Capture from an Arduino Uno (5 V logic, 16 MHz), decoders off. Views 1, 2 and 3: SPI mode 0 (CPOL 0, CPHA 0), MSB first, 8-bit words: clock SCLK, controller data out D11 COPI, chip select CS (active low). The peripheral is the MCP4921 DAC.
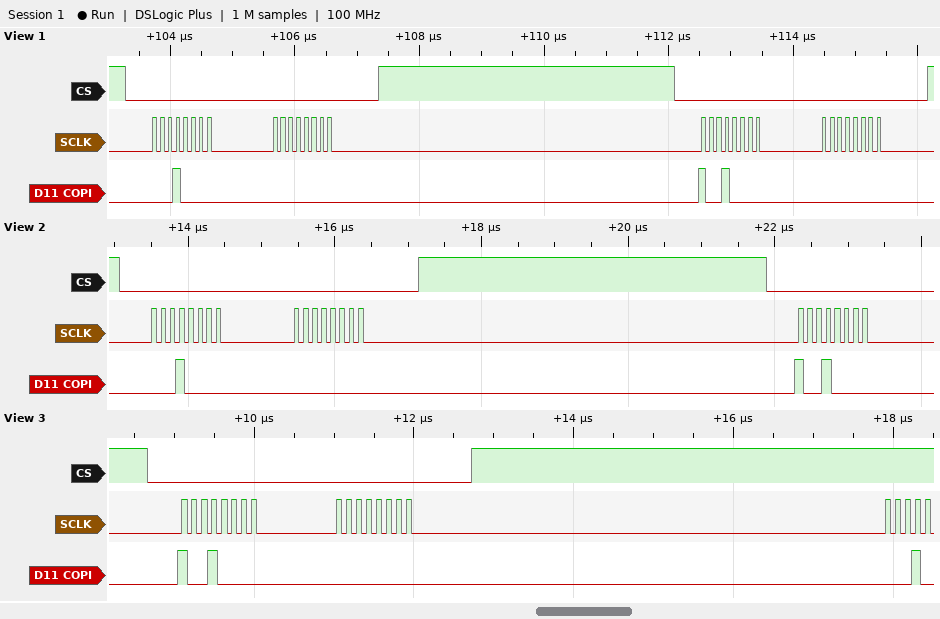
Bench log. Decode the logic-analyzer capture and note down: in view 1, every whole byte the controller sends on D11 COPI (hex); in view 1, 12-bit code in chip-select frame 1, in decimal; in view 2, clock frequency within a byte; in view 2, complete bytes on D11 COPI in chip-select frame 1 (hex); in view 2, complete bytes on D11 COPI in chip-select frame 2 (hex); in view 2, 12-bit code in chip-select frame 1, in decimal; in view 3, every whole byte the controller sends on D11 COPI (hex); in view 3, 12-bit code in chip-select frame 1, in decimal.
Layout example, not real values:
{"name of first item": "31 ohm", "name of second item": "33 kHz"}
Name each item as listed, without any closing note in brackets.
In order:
{"in view 1, every whole byte the controller sends on D11 COPI": "10 00 90 00", "in view 1, 12-bit code in chip-select frame 1, in decimal": "0", "in view 2, clock frequency within a byte": "8 MHz", "in view 2, complete bytes on D11 COPI in chip-select frame 1": "10 00", "in view 2, complete bytes on D11 COPI in chip-select frame 2": "90", "in view 2, 12-bit code in chip-select frame 1, in decimal": "0", "in view 3, every whole byte the controller sends on D11 COPI": "90 00", "in view 3, 12-bit code in chip-select frame 1, in decimal": "0"}
